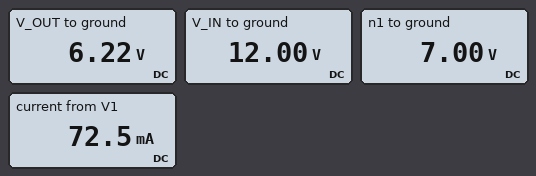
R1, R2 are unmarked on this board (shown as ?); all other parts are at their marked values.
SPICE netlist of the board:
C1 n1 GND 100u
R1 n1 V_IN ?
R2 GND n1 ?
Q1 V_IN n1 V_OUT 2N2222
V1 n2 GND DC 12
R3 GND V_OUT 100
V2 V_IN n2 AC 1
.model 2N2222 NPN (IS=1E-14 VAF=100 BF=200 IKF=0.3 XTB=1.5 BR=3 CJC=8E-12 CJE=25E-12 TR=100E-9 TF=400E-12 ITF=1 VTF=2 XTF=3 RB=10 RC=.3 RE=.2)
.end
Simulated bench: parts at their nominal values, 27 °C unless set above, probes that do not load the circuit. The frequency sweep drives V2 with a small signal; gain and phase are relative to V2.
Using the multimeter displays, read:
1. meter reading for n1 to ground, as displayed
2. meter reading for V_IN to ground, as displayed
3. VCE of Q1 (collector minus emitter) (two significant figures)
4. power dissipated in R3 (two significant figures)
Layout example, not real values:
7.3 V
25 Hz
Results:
7.00 V
12.00 V
5.8 V
390 mW
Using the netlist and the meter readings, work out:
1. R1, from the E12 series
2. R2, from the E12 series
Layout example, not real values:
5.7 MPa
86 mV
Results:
470 Ω
680 Ω
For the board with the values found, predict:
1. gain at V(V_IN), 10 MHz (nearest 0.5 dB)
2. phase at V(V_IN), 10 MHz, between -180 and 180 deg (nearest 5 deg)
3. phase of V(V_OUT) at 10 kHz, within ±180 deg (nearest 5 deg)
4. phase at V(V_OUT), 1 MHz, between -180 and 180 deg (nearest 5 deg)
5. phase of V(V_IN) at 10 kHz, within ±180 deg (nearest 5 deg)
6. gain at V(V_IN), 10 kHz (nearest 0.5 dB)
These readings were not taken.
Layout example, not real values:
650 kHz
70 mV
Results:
0 dB
0 deg
-45 deg
40 deg
0 deg
0 dB
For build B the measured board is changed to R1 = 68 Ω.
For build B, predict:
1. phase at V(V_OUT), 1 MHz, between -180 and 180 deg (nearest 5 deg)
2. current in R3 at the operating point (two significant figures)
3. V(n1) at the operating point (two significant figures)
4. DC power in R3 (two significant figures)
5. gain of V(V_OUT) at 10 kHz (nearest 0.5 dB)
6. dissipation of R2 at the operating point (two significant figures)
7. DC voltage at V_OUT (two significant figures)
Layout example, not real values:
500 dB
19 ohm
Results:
45 deg
100 mA
11 V
1.0 W
-52.5 dB
170 mW
10 V
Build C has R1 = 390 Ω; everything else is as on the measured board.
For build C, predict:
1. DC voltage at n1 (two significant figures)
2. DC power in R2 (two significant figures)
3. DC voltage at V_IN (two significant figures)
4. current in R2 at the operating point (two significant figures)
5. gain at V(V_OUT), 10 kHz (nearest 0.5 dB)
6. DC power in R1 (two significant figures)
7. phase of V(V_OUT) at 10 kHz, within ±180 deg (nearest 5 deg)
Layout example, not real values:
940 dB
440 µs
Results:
7.5 V
83 mW
12 V
11 mA
-65.5 dB
51 mW
-50 deg
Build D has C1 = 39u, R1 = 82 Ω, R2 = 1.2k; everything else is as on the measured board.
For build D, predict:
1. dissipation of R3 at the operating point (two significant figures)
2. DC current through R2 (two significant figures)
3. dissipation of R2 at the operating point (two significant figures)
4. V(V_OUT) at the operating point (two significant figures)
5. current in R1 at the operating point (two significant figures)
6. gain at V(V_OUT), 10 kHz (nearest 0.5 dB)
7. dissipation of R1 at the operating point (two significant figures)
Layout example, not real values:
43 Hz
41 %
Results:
1.1 W
9.3 mA
100 mW
10 V
10 mA
-46.0 dB
8.2 mW
